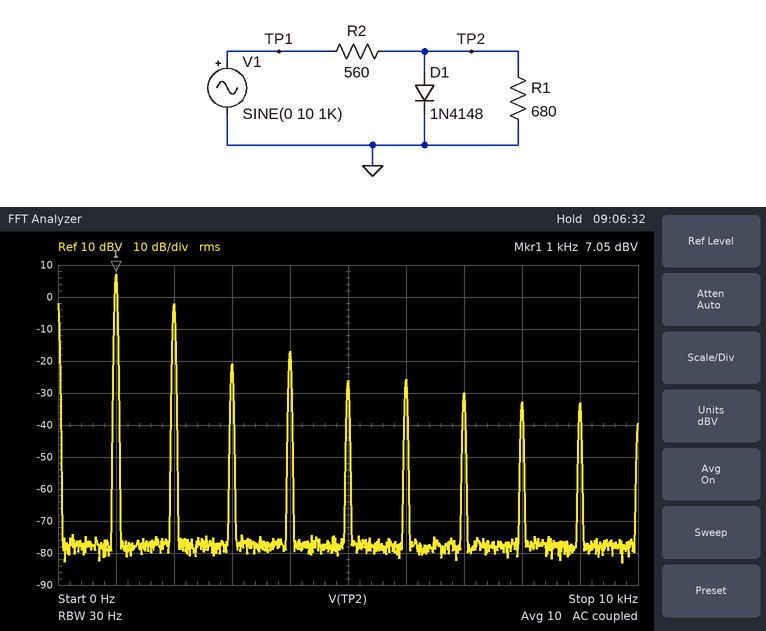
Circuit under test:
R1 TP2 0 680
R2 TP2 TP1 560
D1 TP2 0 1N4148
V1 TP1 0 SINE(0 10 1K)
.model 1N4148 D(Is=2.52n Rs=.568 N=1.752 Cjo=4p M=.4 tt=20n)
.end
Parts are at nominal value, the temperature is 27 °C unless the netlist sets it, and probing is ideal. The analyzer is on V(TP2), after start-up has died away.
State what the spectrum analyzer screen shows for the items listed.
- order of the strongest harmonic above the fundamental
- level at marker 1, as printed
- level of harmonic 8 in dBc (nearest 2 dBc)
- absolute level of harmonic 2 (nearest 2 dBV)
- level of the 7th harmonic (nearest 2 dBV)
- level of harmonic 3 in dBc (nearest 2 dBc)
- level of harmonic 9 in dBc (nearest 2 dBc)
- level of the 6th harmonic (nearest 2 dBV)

2
7.05 dBV
-40 dBc
-2 dBV
-30 dBV
-28 dBc
-40 dBc
-26 dBV
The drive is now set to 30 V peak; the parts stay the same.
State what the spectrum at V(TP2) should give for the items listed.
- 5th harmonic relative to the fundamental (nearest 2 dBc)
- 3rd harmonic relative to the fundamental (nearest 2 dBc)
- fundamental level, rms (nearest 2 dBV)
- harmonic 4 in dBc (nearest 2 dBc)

-40 dBc
-36 dBc
16 dBV
-22 dBc
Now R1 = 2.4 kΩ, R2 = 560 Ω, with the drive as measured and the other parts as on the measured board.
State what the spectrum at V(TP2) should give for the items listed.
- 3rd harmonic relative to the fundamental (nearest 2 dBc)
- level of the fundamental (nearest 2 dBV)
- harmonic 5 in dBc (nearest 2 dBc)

-30 dBc
10 dBV
-36 dBc
